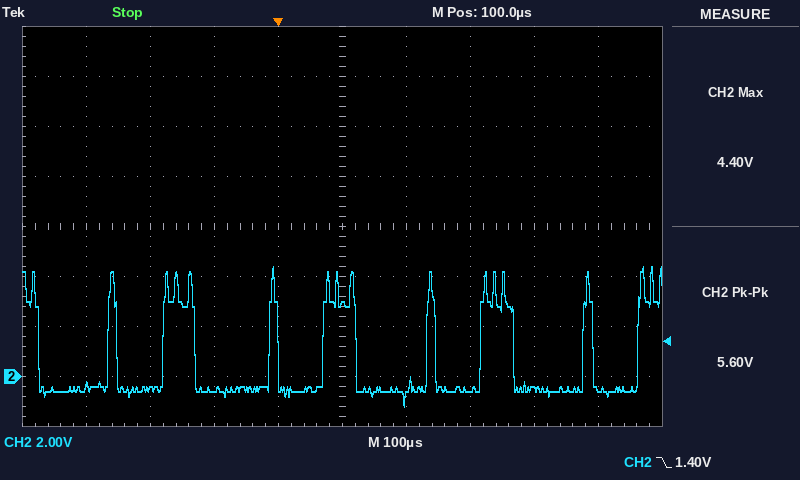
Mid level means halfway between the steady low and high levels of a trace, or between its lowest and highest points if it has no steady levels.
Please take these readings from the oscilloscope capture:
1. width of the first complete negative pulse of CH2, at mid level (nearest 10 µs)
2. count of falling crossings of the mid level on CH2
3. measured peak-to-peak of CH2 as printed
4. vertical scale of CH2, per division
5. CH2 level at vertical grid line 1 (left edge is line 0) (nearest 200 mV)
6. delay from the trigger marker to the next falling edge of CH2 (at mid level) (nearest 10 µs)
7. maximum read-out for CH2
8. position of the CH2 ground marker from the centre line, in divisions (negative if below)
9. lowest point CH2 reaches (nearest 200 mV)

110 µs
8
5.60 V
2 V
-400 mV
120 µs
4.40 V
-3.0 div
-1.2 V
